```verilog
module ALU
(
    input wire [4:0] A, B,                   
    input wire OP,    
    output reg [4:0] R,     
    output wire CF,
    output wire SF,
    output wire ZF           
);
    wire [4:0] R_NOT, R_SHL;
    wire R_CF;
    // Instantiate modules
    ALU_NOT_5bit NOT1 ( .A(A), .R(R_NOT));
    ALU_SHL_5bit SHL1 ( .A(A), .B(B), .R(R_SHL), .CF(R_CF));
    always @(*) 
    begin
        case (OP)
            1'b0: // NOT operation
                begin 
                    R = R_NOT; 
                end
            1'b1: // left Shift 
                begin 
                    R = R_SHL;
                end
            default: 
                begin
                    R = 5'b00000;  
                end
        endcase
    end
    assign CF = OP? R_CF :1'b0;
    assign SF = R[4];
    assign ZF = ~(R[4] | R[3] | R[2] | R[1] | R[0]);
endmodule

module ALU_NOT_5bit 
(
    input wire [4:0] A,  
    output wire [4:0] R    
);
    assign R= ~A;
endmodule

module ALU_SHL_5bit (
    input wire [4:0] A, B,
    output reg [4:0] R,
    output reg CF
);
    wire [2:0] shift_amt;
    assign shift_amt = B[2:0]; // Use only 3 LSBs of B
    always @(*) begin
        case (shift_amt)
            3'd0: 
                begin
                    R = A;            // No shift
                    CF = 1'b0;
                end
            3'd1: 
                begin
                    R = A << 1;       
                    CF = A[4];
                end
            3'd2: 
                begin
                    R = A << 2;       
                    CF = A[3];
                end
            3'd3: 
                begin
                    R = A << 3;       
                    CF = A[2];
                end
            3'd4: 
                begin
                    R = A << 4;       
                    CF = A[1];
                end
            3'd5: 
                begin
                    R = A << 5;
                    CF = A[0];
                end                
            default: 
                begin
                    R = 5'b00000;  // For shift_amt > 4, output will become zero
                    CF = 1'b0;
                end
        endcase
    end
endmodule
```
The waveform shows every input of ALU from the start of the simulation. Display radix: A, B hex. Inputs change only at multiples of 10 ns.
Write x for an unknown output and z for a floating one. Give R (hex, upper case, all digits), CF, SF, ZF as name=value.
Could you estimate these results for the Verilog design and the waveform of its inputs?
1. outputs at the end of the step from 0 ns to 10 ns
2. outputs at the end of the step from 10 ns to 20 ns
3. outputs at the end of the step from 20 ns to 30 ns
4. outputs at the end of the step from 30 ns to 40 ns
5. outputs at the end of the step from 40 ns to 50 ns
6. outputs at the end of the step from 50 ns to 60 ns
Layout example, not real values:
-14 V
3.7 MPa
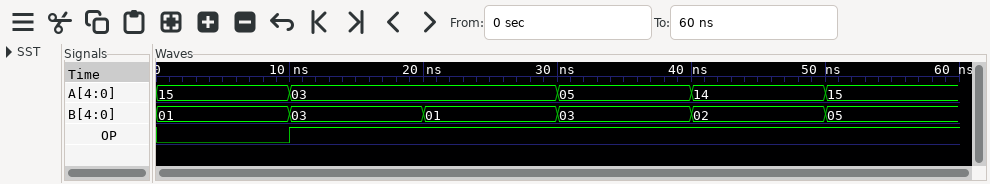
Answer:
R=0A, CF=0, SF=0, ZF=0
R=18, CF=0, SF=1, ZF=0
R=06, CF=0, SF=0, ZF=0
R=08, CF=1, SF=0, ZF=0
R=10, CF=0, SF=1, ZF=0
R=00, CF=1, SF=0, ZF=1
